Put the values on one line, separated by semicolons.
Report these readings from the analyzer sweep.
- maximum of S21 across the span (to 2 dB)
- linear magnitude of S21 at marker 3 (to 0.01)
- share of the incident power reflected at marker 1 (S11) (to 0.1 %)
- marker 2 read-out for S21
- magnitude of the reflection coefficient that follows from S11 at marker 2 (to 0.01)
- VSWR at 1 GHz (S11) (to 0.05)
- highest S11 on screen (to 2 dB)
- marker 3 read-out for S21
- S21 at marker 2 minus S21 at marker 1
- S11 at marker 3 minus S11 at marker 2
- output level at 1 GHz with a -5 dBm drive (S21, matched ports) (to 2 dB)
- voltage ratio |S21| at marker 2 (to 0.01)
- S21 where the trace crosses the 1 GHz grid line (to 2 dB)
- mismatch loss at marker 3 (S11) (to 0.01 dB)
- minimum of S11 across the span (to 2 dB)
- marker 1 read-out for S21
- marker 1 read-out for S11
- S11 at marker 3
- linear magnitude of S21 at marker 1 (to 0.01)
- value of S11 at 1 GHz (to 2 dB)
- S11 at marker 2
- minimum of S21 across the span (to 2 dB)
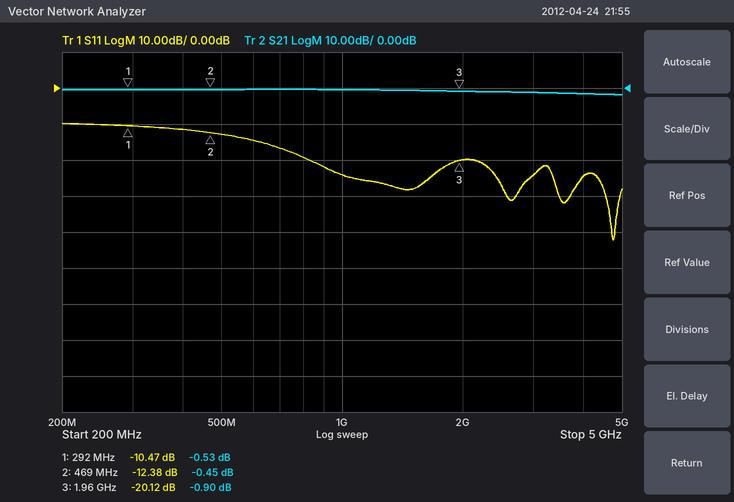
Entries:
0 dB; 0.90; 9.0 %; -0.45 dB; 0.24; 1.15; -10 dB; -0.90 dB; 0.08 dB; -7.74 dB; -6 dBm; 0.95; 0 dB; 0.04 dB; -42 dB; -0.53 dB; -10.47 dB; -20.12 dB; 0.94; -24 dB; -12.38 dB; -2 dB
